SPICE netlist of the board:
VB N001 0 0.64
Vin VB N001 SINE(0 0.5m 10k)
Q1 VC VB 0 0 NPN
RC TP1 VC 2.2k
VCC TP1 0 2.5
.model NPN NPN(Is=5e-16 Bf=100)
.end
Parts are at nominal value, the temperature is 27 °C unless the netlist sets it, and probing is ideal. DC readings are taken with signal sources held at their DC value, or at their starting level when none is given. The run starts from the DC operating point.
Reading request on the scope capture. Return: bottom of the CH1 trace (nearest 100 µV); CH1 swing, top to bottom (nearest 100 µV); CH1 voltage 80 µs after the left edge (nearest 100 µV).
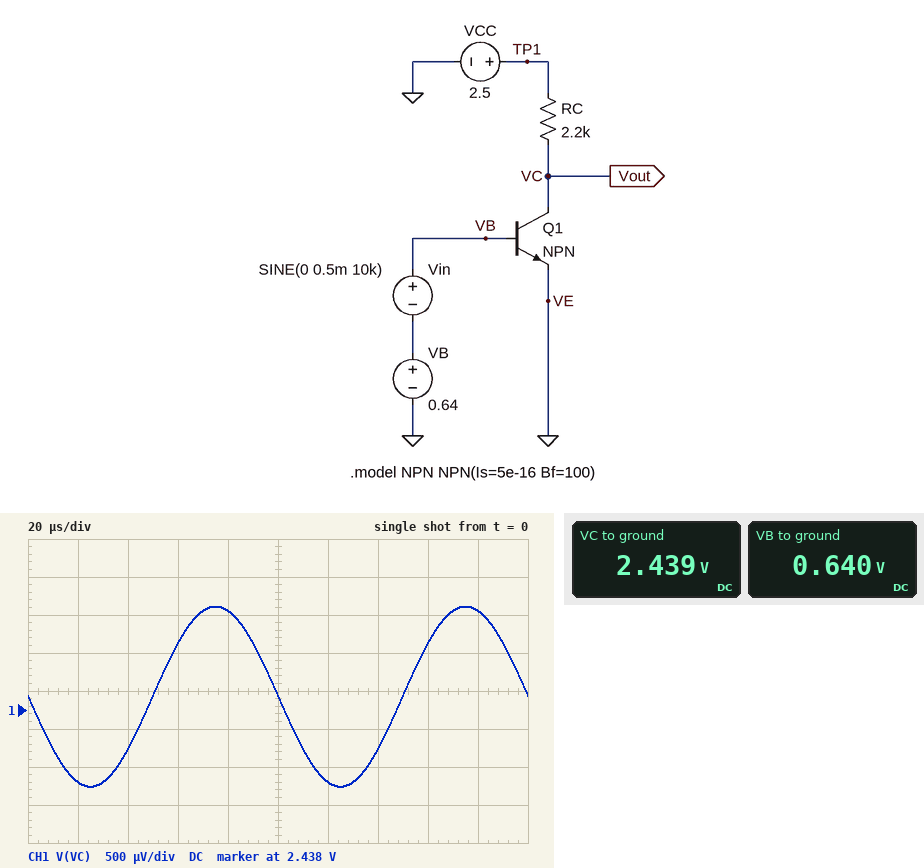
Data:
2.4375 V
2.4 mV
2.4398 V
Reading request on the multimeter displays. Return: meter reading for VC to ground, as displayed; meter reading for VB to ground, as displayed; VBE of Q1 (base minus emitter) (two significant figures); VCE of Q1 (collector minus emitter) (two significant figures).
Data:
2.439 V
0.640 V
640 mV
2.4 V
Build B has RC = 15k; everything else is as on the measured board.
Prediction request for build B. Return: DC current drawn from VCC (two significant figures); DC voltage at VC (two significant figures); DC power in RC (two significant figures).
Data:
28 µA
2.1 V
12 µW
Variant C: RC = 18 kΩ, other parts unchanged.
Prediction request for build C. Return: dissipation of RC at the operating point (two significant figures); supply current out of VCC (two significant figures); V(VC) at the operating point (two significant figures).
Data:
14 µW
28 µA
2.0 V
